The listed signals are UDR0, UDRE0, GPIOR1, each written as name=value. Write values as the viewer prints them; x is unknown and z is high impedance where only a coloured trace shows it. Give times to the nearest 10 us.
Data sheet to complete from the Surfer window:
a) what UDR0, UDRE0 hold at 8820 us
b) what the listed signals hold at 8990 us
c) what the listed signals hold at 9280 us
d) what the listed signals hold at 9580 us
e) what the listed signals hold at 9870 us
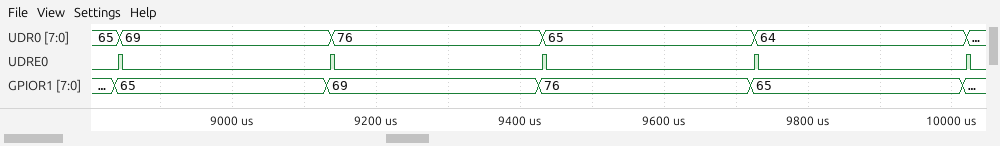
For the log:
UDR0=65, UDRE0=0
UDR0=69, UDRE0=0, GPIOR1=65
UDR0=76, UDRE0=0, GPIOR1=69
UDR0=65, UDRE0=0, GPIOR1=76
UDR0=64, UDRE0=0, GPIOR1=65
